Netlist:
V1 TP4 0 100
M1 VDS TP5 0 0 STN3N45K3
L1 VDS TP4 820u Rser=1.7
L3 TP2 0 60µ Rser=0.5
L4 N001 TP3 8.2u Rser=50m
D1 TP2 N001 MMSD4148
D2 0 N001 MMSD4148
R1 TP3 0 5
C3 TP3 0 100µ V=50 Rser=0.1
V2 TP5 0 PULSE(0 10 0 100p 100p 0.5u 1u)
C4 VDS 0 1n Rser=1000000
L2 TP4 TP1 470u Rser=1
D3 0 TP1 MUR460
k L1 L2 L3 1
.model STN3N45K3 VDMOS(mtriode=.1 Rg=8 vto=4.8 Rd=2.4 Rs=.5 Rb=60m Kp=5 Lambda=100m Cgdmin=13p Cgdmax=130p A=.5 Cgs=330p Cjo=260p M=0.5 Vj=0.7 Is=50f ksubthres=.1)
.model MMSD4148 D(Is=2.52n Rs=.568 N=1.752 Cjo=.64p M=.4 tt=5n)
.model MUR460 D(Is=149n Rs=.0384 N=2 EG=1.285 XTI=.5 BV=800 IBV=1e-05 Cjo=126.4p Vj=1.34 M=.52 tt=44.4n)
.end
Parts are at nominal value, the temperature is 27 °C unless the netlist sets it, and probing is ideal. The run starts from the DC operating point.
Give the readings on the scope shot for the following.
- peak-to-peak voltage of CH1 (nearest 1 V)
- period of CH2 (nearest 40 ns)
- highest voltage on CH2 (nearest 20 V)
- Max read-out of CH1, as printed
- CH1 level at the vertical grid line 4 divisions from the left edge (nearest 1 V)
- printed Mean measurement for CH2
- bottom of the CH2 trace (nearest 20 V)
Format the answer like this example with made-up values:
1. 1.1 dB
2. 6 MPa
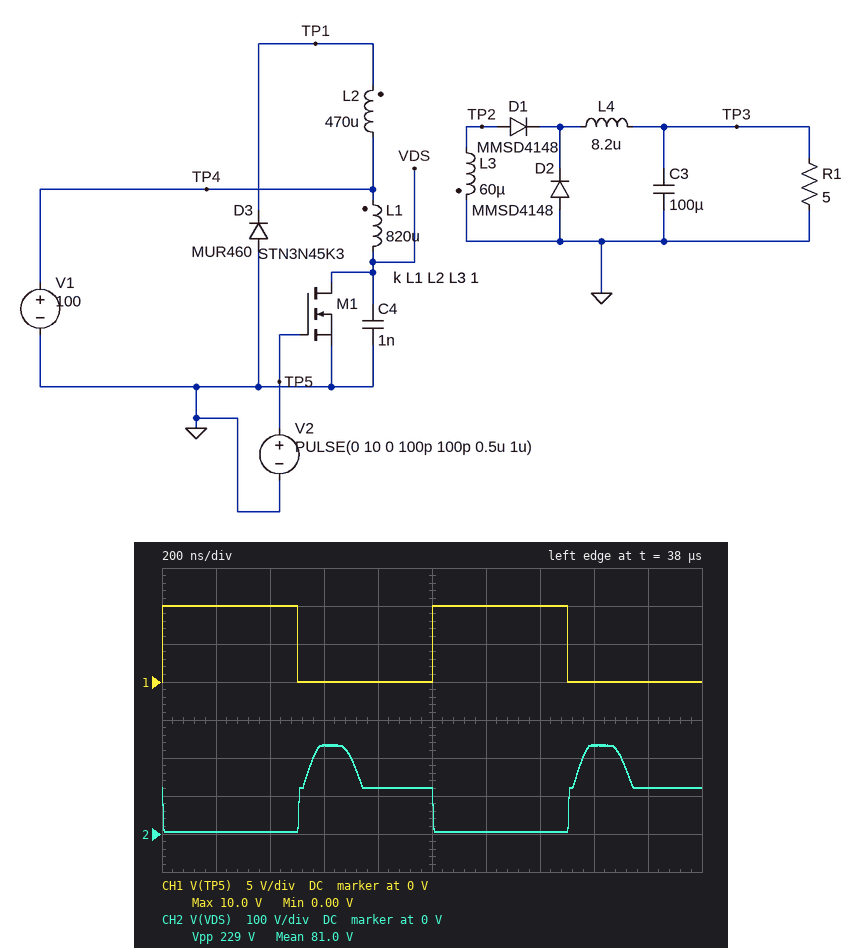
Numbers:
1. 10 V
2. 1.00 µs
3. 240 V
4. 10.0 V
5. 0 V
6. 81.0 V
7. 0 V
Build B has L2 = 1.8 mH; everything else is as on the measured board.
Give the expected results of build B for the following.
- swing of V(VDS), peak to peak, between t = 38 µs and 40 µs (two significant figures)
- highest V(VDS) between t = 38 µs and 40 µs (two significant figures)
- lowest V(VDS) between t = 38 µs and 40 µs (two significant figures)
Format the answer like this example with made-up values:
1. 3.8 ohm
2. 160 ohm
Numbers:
1. 160 V
2. 170 V
3. 4.3 V
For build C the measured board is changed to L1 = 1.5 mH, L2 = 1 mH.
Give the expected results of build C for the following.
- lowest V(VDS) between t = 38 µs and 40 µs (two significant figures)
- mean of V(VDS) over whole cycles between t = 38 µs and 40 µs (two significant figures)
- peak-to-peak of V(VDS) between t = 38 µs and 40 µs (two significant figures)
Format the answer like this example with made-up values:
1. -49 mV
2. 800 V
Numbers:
1. 2.1 V
2. 81 V
3. 220 V
